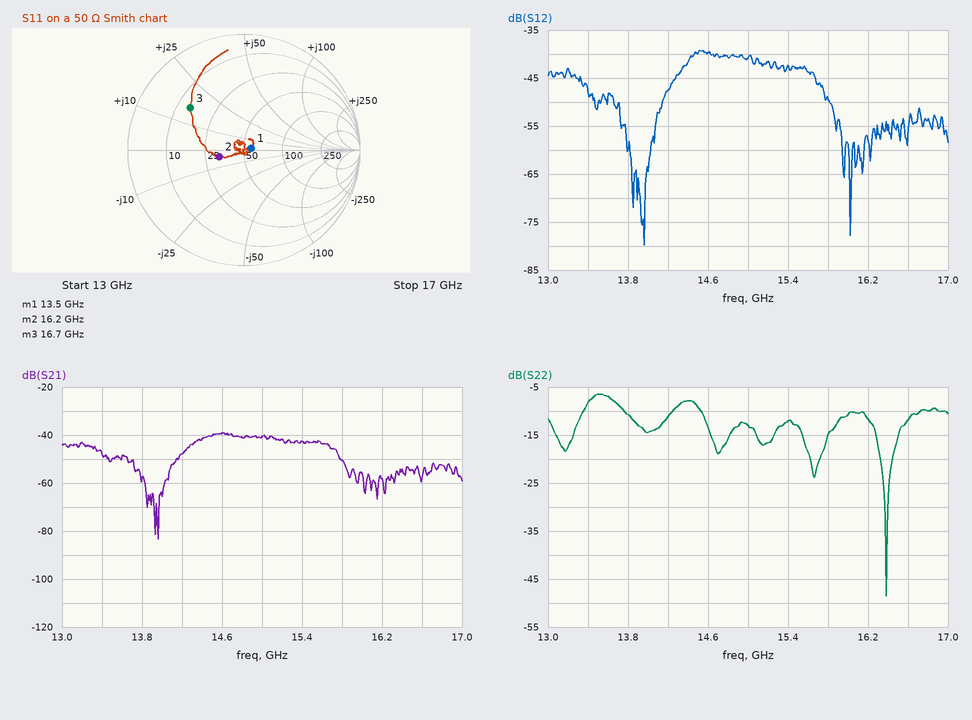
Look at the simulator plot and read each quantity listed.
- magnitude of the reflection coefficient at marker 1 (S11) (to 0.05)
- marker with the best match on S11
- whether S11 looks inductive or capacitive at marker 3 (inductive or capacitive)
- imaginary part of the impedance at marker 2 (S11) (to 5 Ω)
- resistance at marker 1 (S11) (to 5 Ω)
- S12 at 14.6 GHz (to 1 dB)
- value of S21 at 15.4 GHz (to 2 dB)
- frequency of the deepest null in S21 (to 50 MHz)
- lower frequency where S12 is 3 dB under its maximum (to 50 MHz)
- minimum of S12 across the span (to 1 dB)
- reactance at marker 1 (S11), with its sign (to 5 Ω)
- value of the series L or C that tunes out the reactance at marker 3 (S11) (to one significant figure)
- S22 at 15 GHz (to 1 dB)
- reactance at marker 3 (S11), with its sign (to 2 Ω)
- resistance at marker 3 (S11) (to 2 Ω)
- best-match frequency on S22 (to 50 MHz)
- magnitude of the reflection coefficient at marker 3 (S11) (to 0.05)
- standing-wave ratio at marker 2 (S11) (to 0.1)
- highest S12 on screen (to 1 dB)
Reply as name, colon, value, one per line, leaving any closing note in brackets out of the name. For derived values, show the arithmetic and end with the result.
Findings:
magnitude of the reflection coefficient at marker 1 (S11): 0.05
marker with the best match on S11: marker 1
whether S11 looks inductive or capacitive at marker 3: inductive
imaginary part of the impedance at marker 2 (S11): -5 Ω
resistance at marker 1 (S11): 55 Ω
S12 at 14.6 GHz: -40 dB
value of S21 at 15.4 GHz: -42 dB
frequency of the deepest null in S21: 13.95 GHz
lower frequency where S12 is 3 dB under its maximum: 14.40 GHz
minimum of S12 across the span: -80 dB
reactance at marker 1 (S11), with its sign: 0 Ω
value of the series L or C that tunes out the reactance at marker 3 (S11): C = 1/(2π × 16.7 GHz × 16 Ω) ≈ 596 fF, so 600 fF to one significant figure
S22 at 15 GHz: -13 dB
reactance at marker 3 (S11), with its sign: +16 Ω
resistance at marker 3 (S11): 14 Ω
best-match frequency on S22: 16.40 GHz
magnitude of the reflection coefficient at marker 3 (S11): 0.60
standing-wave ratio at marker 2 (S11): 1.6
highest S12 on screen: -39 dB
